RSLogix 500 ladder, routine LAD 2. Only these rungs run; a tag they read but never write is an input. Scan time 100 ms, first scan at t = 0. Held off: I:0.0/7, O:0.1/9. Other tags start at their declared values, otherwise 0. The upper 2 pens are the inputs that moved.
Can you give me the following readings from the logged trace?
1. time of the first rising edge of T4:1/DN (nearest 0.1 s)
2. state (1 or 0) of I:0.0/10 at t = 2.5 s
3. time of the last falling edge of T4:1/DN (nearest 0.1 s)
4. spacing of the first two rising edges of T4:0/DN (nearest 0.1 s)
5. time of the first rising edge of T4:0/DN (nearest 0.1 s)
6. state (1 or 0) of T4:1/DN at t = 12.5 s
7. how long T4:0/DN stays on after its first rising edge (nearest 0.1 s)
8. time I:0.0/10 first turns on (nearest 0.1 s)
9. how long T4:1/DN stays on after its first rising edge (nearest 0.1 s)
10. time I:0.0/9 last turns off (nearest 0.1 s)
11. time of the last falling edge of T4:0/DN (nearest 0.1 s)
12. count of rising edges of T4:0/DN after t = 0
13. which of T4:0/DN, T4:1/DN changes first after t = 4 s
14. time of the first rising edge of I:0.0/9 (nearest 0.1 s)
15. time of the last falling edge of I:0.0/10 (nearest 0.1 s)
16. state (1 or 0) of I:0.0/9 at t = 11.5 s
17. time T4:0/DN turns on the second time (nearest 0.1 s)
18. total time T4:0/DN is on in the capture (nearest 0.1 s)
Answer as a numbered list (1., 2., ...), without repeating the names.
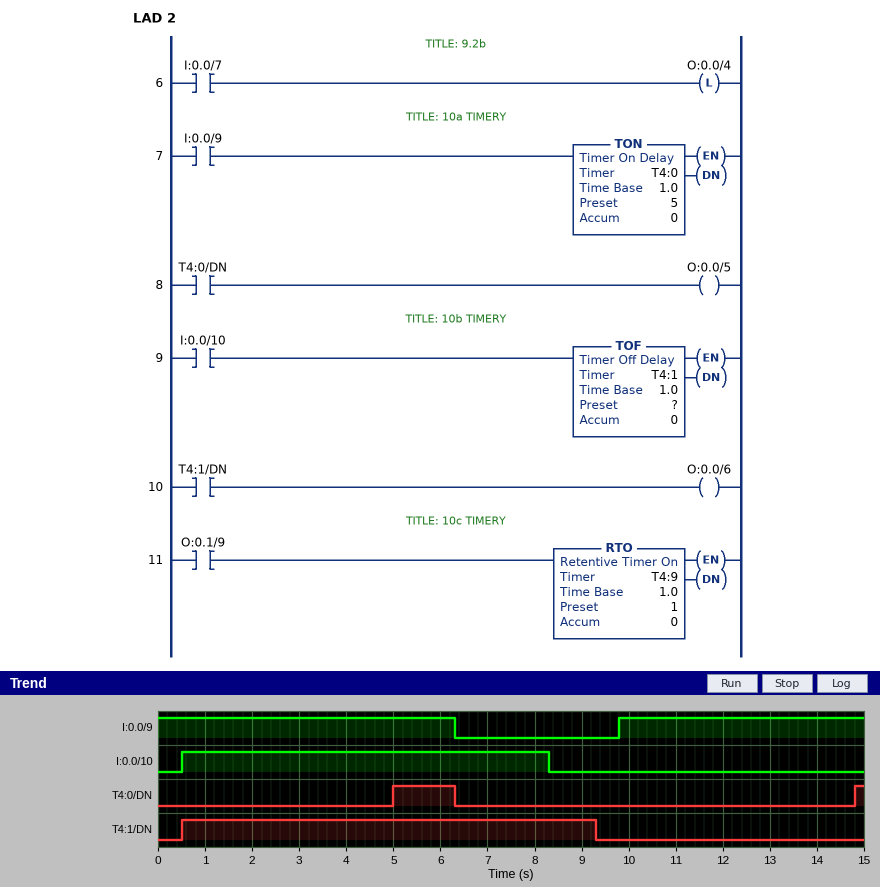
1. 0.5 s
2. 1
3. 9.3 s
4. 9.8 s
5. 5.0 s
6. 0
7. 1.3 s
8. 0.5 s
9. 8.8 s
10. 6.3 s
11. 6.3 s
12. 2
13. T4:0/DN
14. 9.8 s
15. 8.3 s
16. 1
17. 14.8 s
18. 1.5 s
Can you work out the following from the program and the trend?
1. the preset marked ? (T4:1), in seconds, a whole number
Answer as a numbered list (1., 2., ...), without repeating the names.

1. 1 s
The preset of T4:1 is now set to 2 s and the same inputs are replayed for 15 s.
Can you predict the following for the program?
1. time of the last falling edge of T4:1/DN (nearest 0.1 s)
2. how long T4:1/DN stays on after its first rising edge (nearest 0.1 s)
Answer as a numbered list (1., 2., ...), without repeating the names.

1. 10.3 s
2. 9.8 s
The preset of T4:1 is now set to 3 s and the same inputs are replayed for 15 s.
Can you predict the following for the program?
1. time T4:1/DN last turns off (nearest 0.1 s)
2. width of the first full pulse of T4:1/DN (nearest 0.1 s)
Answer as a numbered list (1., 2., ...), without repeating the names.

1. 11.3 s
2. 10.8 s
